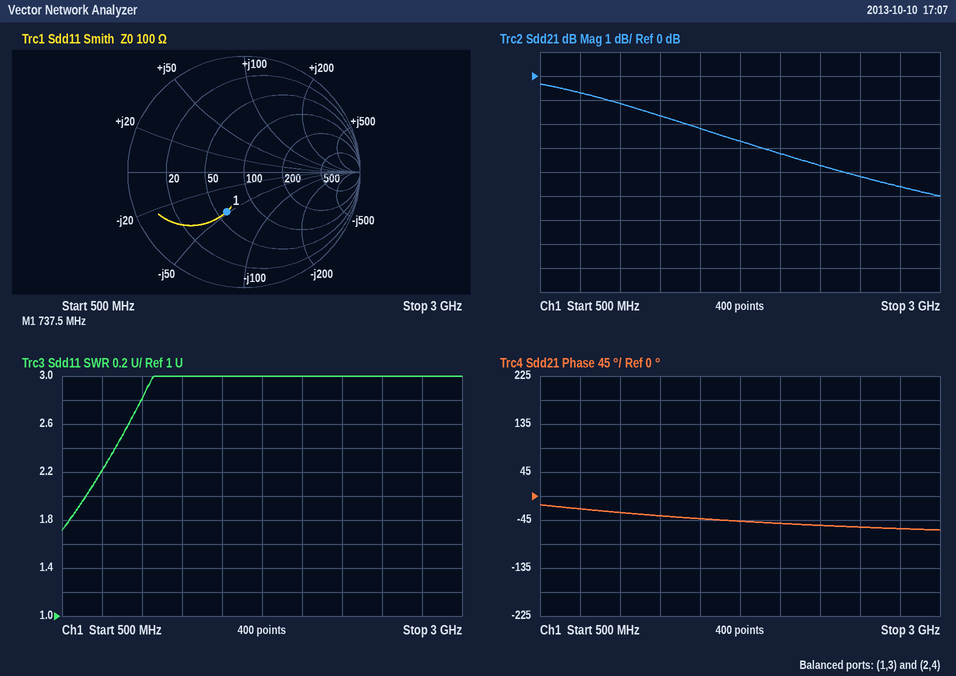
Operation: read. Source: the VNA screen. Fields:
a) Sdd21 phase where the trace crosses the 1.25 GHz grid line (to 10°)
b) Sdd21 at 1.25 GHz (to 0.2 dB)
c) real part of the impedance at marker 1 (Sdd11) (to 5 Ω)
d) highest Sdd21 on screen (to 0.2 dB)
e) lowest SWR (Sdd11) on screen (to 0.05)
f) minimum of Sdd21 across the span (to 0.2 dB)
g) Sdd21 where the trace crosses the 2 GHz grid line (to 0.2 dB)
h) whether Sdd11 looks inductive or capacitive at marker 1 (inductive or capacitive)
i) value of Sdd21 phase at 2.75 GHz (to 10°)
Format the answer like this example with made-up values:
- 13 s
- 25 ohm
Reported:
- -40°
- -1.6 dB
- 60 Ω
- -0.4 dB
- 1.70
- -5.0 dB
- -3.2 dB
- capacitive
- -60°
